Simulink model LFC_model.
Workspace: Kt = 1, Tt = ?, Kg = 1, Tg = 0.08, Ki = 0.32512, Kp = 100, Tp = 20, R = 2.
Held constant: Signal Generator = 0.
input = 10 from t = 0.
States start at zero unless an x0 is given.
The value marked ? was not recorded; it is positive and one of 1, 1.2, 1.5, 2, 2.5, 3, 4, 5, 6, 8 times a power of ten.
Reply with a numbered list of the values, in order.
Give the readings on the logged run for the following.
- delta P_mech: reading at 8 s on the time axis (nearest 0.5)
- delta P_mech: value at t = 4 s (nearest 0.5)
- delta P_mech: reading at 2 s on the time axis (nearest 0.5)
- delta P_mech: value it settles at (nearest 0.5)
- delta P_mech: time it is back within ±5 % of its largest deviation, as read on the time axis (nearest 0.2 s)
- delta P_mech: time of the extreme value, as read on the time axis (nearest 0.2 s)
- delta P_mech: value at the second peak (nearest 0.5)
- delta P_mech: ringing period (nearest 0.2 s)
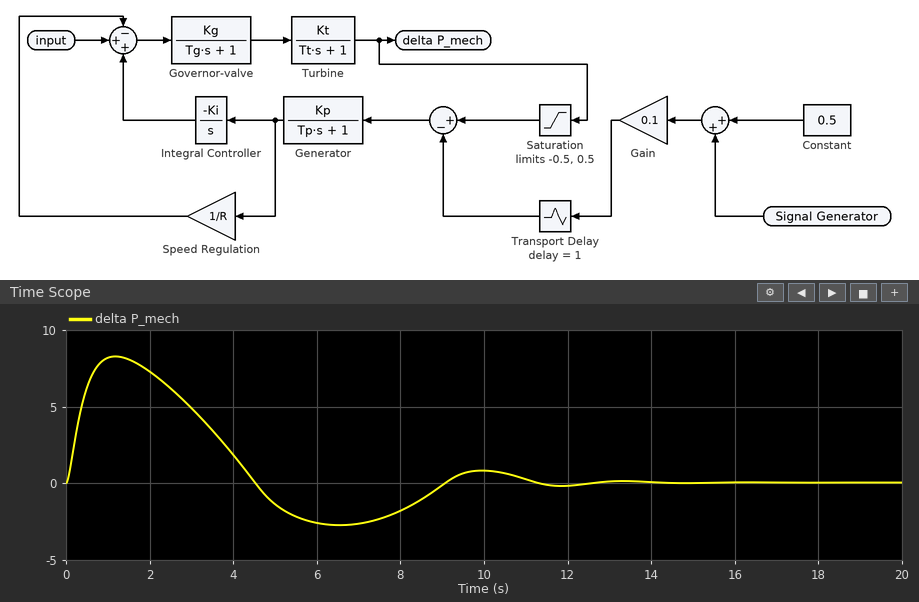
1. -2.0
2. 2.0
3. 7.5
4. 0.0
5. 10.8 s
6. 1.2 s
7. 1.0
8. 8.8 s
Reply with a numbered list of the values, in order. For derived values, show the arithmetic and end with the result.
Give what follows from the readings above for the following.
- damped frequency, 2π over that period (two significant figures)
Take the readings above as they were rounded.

1. 2π / 8.8 = 0.71 rad/s
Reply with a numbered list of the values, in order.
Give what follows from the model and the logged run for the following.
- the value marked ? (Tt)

1. 0.4
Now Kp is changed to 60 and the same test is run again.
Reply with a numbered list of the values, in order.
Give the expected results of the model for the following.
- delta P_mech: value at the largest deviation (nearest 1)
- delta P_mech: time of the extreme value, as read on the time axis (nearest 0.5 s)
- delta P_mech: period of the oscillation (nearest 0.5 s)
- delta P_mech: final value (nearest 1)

1. 9
2. 1.5 s
3. 12.5 s
4. 0
